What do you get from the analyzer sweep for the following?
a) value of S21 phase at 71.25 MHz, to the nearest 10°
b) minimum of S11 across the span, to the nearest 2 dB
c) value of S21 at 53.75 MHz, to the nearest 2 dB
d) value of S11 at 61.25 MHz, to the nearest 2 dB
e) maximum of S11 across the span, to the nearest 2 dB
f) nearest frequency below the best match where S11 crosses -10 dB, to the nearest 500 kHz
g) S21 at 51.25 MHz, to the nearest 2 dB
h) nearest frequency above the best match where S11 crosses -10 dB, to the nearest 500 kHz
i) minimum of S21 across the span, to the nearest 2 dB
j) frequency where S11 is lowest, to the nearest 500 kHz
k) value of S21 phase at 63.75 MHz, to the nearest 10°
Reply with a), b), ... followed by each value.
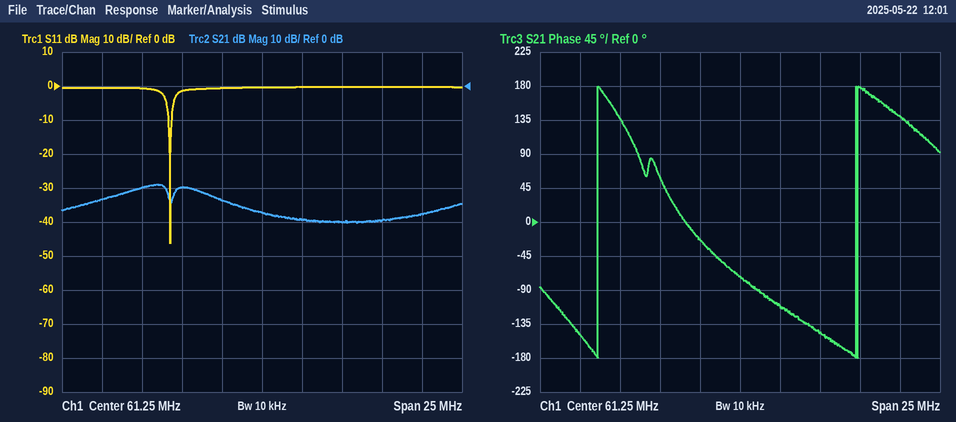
a) 140°
b) -46 dB
c) -30 dB
d) 0 dB
e) 0 dB
f) 55.5 MHz
g) -34 dB
h) 55.5 MHz
i) -40 dB
j) 55.5 MHz
k) -110°
